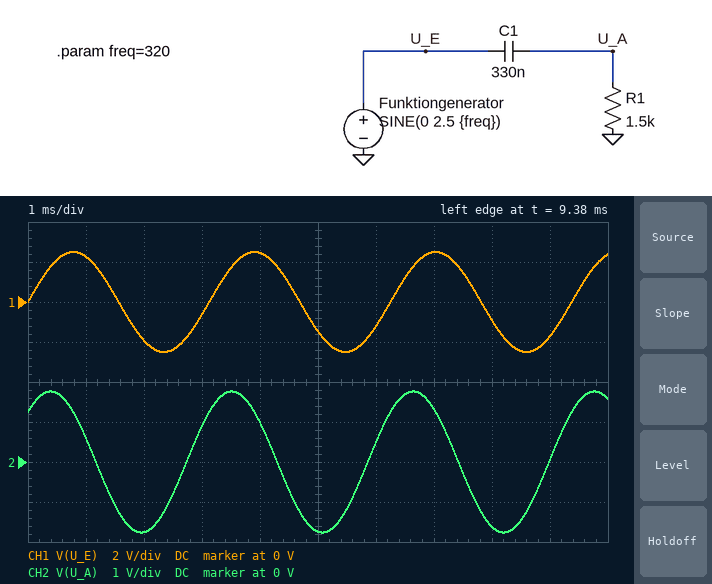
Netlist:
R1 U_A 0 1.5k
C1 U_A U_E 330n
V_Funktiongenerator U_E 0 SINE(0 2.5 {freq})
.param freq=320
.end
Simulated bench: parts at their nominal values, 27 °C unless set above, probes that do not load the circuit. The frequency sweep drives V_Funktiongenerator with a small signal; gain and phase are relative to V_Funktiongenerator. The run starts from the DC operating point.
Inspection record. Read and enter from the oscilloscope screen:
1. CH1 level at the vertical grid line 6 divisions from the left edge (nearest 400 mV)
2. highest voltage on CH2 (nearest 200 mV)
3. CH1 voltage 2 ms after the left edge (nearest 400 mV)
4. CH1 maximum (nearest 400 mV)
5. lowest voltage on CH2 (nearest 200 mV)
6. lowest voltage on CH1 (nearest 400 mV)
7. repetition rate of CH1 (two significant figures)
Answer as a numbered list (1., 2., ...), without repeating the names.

1. -1.2 V
2. 1.8 V
3. -2.0 V
4. 2.4 V
5. -1.8 V
6. -2.4 V
7. 320 Hz
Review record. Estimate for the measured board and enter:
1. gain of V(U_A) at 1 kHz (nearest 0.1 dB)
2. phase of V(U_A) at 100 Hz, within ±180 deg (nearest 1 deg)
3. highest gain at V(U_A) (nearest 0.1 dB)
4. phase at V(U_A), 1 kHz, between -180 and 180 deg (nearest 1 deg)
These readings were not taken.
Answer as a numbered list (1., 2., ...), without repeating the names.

1. -0.4 dB
2. 73 deg
3. 0 dB
4. 18 deg
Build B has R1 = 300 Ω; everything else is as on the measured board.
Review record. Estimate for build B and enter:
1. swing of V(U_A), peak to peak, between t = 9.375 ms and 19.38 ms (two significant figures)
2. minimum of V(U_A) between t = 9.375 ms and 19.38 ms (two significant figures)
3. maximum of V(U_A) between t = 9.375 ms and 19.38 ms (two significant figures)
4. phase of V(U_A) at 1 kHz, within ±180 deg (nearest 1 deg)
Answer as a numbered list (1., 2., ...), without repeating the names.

1. 980 mV
2. -490 mV
3. 490 mV
4. 58 deg
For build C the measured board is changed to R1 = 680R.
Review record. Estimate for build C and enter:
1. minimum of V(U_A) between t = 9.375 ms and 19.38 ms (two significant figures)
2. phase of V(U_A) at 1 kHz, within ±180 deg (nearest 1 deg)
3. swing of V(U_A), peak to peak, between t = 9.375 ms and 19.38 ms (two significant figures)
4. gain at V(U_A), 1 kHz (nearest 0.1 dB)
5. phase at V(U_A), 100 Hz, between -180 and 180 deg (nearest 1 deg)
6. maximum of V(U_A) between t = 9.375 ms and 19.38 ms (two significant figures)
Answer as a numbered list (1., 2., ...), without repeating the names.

1. -1.0 V
2. 35 deg
3. 2.1 V
4. -1.8 dB
5. 82 deg
6. 1.0 V
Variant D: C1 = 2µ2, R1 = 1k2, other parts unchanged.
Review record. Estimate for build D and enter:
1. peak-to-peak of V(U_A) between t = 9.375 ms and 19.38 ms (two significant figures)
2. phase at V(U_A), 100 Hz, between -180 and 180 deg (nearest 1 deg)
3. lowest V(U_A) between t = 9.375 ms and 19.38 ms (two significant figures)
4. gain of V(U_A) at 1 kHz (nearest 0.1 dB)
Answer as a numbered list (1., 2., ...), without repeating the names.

1. 4.9 V
2. 31 deg
3. -2.5 V
4. 0 dB
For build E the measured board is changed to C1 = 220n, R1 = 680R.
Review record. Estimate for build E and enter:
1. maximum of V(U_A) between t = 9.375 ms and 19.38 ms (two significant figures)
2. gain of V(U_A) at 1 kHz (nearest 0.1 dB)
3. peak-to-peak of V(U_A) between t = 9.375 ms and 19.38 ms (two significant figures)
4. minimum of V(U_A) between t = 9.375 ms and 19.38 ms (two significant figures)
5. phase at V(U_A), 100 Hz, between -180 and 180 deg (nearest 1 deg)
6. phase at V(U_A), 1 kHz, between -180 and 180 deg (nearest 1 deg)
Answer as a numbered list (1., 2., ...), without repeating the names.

1. 720 mV
2. -3.3 dB
3. 1.4 V
4. -720 mV
5. 85 deg
6. 47 deg
